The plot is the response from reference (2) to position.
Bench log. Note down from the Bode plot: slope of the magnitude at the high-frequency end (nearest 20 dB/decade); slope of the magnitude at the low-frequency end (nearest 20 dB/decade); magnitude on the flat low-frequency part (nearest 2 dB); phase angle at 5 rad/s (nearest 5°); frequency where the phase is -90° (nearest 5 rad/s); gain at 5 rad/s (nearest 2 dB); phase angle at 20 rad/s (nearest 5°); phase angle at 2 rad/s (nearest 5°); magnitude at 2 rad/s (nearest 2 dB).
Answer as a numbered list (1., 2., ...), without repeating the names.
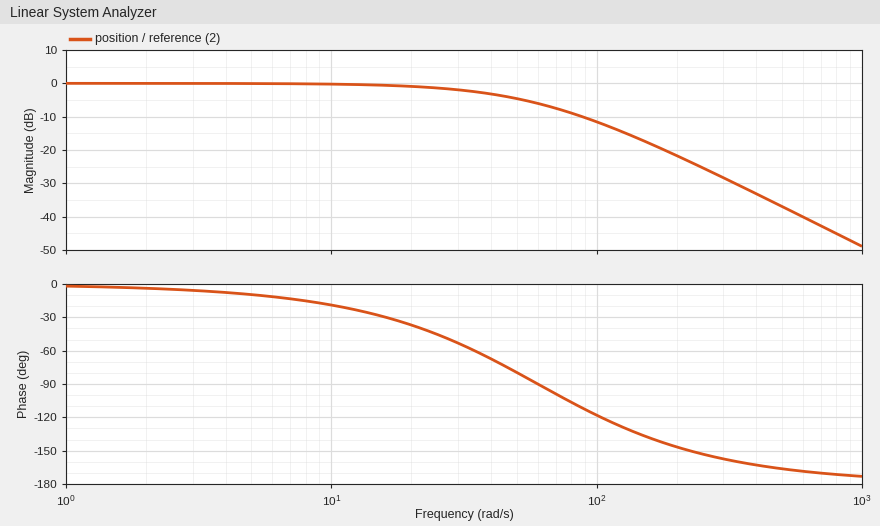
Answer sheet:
1. -40 dB/decade
2. 0 dB/decade
3. 0 dB
4. -10°
5. 60 rad/s
6. 0 dB
7. -35°
8. -5°
9. 0 dB
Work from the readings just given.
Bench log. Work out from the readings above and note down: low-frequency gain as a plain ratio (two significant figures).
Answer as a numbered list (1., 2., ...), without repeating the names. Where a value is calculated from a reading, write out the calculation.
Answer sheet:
1. 10^(0 / 20) = 1.0
